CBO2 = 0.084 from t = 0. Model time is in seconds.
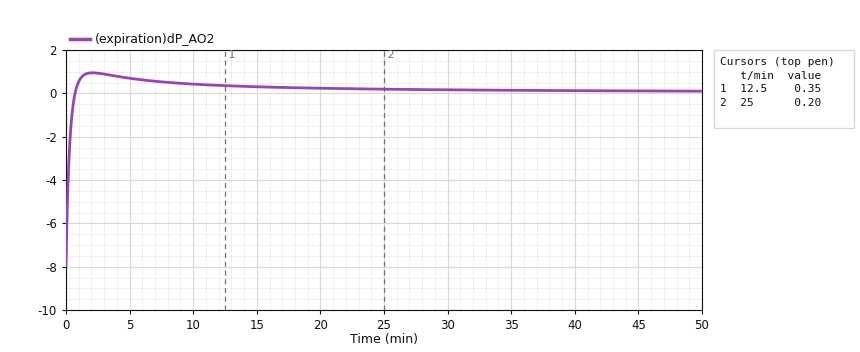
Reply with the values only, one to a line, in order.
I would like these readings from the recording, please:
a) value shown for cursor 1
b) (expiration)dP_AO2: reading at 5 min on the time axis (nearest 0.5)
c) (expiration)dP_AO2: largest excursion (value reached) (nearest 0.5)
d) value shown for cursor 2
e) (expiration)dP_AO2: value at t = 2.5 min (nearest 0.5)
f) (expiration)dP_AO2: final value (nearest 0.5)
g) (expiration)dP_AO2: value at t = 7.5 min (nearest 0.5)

0.35
0.5
1.0
0.20
1.0
0.0
0.5
